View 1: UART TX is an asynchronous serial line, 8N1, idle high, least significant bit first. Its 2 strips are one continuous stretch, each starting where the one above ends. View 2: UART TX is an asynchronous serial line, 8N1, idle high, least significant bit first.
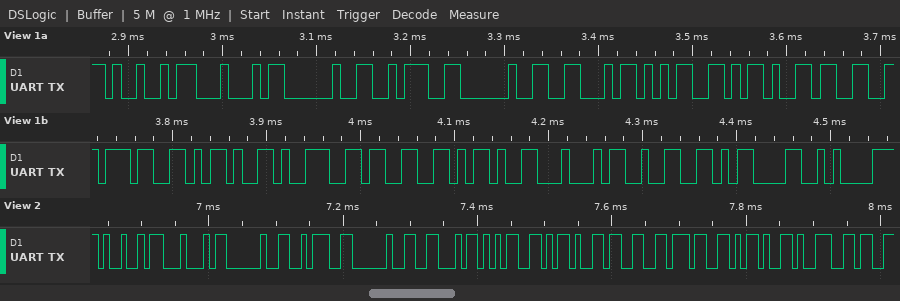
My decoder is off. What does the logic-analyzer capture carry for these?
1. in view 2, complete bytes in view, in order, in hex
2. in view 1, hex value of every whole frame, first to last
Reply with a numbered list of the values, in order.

1. 49 44 20 3A 20 46 35 2D 33 37 2D 39
2. 49 44 20 3A 20 46 35 2D 33 37 2D 39 33 2D 44 32 0D 0A
